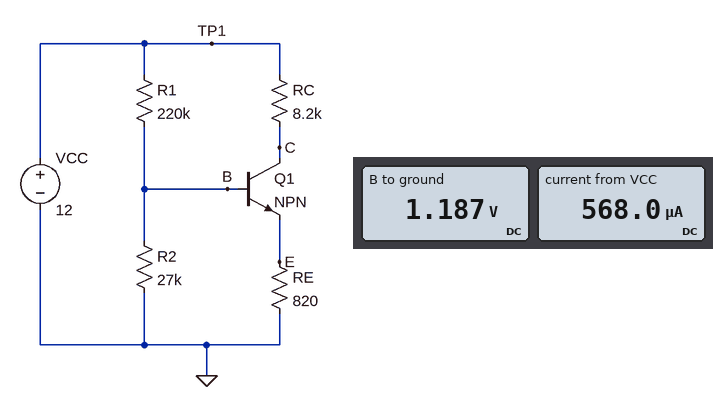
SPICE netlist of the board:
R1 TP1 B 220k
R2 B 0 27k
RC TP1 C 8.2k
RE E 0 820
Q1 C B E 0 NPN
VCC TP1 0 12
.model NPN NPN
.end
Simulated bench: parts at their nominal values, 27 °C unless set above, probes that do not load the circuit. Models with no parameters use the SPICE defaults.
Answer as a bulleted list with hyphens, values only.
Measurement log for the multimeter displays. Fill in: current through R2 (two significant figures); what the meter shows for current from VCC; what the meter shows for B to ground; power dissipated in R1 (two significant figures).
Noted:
- 44 µA
- 568.0 µA
- 1.187 V
- 530 µW
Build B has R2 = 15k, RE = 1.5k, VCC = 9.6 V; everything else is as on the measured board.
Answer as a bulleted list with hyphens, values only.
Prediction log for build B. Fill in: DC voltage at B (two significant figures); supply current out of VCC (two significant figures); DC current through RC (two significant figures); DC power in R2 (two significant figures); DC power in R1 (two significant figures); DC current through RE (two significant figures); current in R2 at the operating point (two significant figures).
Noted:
- 610 mV
- 43 µA
- 1.7 µA
- 25 µW
- 370 µW
- 1.8 µA
- 41 µA
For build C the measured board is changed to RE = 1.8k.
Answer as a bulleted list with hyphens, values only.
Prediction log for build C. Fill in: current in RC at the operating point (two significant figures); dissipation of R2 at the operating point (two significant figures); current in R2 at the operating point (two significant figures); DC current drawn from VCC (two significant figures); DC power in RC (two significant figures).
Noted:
- 280 µA
- 57 µW
- 46 µA
- 330 µA
- 630 µW
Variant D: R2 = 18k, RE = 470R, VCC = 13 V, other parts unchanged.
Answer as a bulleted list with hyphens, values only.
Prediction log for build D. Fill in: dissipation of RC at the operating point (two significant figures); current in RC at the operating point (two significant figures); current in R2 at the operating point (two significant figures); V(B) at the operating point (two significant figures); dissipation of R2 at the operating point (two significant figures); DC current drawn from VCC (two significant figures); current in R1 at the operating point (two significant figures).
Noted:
- 1.1 mW
- 370 µA
- 51 µA
- 920 mV
- 47 µW
- 420 µA
- 55 µA
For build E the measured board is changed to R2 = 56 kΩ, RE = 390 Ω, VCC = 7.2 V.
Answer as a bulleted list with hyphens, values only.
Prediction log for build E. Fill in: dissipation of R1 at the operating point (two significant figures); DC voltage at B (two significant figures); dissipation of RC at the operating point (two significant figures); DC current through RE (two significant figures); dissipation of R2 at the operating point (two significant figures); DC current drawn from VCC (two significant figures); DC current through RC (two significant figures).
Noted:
- 170 µW
- 1.1 V
- 5.4 mW
- 820 µA
- 21 µW
- 840 µA
- 810 µA
